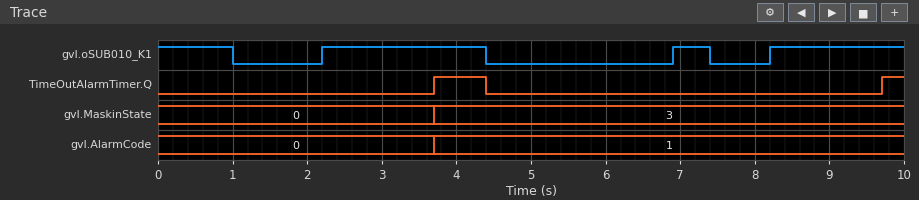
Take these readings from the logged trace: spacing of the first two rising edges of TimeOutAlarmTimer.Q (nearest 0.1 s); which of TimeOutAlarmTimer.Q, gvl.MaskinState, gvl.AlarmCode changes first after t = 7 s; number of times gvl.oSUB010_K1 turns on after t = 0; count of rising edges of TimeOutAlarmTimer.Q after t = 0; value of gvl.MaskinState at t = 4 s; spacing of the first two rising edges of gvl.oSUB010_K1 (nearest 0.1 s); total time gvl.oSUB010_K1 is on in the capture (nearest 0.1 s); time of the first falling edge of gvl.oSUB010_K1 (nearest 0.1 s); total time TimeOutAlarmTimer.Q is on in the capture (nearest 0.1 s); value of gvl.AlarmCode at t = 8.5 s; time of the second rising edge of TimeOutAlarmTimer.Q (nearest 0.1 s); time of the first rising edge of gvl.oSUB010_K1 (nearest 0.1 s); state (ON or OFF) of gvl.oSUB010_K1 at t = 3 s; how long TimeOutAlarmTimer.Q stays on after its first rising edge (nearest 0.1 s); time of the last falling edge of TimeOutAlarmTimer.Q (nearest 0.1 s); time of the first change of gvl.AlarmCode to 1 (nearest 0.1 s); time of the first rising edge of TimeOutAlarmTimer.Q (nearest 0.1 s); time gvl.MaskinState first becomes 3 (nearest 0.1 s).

6.0 s
TimeOutAlarmTimer.Q
3
2
3
4.7 s
5.5 s
1.0 s
1.0 s
1
9.7 s
2.2 s
ON
0.7 s
4.4 s
3.7 s
3.7 s
3.7 s
